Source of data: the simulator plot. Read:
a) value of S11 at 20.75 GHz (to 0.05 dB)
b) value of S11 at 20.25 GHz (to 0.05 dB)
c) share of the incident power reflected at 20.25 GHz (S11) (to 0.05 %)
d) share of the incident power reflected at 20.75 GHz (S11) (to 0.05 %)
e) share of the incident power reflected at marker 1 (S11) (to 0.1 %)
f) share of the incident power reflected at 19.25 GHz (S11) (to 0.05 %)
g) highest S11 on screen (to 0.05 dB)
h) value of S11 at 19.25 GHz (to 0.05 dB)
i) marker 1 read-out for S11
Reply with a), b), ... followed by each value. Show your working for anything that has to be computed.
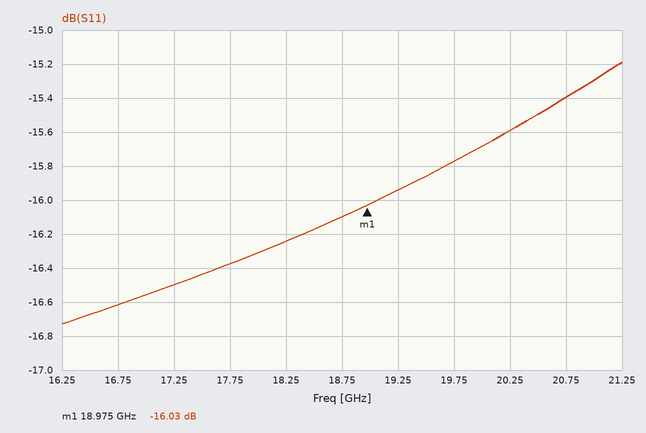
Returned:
a) -15.40 dB
b) -15.60 dB
c) 10^(-15.6/10) ≈ 2.75 %
d) 10^(-15.4/10) ≈ 2.88 %, so 2.90 % to the nearest 0.05 %
e) 10^(-16.03/10) ≈ 2.5 %
f) 10^(-15.95/10) ≈ 2.54 %, so 2.55 % to the nearest 0.05 %
g) -15.20 dB
h) -15.95 dB
i) -16.03 dB
